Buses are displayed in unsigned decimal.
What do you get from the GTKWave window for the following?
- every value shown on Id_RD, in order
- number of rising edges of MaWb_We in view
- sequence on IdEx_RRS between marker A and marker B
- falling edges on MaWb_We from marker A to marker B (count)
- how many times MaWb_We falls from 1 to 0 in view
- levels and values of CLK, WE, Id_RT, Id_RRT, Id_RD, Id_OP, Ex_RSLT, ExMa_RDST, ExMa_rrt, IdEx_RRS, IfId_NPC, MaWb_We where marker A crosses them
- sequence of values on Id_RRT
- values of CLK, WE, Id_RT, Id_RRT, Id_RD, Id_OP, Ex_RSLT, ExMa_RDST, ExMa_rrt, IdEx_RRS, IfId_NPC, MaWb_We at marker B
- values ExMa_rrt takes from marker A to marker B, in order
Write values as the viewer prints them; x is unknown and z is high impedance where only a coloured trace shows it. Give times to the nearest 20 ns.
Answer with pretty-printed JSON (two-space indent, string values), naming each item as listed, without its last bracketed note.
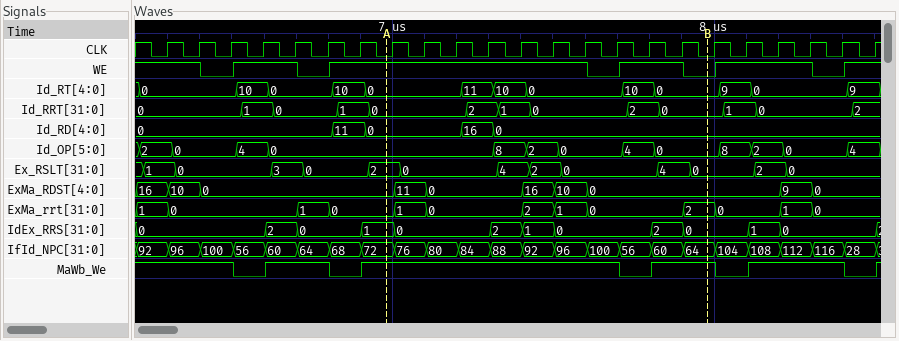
{
  "every value shown on Id_RD, in order": "0, 11, 0, 16, 0",
  "number of rising edges of MaWb_We in view": "5",
  "sequence on IdEx_RRS between marker A and marker B": "1, 0, 2, 1, 0, 2, 0",
  "falling edges on MaWb_We from marker A to marker B": "1",
  "how many times MaWb_We falls from 1 to 0 in view": "5",
  "levels and values of CLK, WE, Id_RT, Id_RRT, Id_RD, Id_OP, Ex_RSLT, ExMa_RDST, ExMa_rrt, IdEx_RRS, IfId_NPC, MaWb_We where marker A crosses them": "CLK=0, WE=1, Id_RT=0, Id_RRT=0, Id_RD=0, Id_OP=0, Ex_RSLT=2, ExMa_RDST=0, ExMa_rrt=0, IdEx_RRS=1, IfId_NPC=72, MaWb_We=1",
  "sequence of values on Id_RRT": "0, 1, 0, 1, 0, 2, 1, 0, 2, 0, 1, 0, 2",
  "values of CLK, WE, Id_RT, Id_RRT, Id_RD, Id_OP, Ex_RSLT, ExMa_RDST, ExMa_rrt, IdEx_RRS, IfId_NPC, MaWb_We at marker B": "CLK=0, WE=0, Id_RT=0, Id_RRT=0, Id_RD=0, Id_OP=0, Ex_RSLT=0, ExMa_RDST=0, ExMa_rrt=2, IdEx_RRS=0, IfId_NPC=64, MaWb_We=1",
  "values ExMa_rrt takes from marker A to marker B, in order": "0, 1, 0, 2, 1, 0, 2"
}
